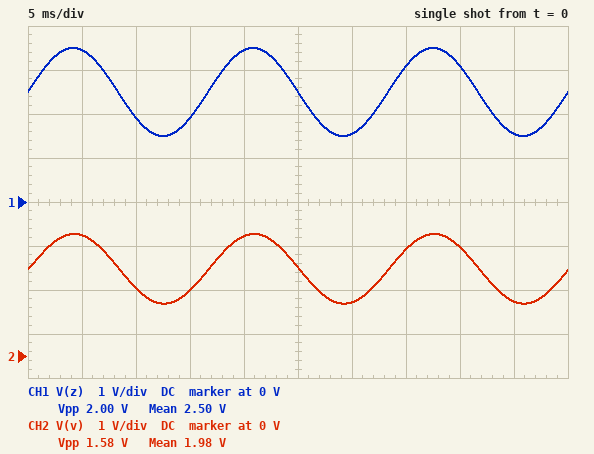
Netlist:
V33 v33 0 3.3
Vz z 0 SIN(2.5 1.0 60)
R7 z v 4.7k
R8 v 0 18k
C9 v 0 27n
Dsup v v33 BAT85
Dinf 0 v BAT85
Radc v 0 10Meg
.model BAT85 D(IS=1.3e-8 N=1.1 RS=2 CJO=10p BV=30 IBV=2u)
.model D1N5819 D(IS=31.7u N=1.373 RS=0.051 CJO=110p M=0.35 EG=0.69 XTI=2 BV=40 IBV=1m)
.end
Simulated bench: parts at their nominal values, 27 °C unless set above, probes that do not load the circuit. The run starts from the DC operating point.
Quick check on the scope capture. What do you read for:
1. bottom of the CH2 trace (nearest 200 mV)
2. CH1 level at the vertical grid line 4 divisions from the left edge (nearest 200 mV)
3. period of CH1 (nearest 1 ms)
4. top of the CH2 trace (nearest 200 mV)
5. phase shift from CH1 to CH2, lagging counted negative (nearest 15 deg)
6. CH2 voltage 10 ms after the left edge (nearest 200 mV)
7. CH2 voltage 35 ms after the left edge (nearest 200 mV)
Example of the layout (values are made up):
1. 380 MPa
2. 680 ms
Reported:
1. 1.2 V
2. 3.4 V
3. 17 ms
4. 2.8 V
5. 0 deg
6. 1.6 V
7. 2.4 V
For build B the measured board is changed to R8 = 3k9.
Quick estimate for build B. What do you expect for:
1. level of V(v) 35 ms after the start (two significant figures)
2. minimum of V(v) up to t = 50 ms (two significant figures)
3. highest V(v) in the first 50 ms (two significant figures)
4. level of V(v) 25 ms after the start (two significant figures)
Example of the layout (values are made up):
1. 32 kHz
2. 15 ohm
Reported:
1. 1.4 V
2. 680 mV
3. 1.6 V
4. 1.1 V
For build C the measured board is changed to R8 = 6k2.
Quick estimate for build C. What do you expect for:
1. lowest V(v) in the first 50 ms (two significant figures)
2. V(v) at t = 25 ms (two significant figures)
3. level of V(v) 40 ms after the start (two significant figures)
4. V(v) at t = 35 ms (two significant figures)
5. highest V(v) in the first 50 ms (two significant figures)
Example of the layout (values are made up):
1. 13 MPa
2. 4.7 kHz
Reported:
1. 850 mV
2. 1.4 V
3. 1.8 V
4. 1.7 V
5. 2.0 V
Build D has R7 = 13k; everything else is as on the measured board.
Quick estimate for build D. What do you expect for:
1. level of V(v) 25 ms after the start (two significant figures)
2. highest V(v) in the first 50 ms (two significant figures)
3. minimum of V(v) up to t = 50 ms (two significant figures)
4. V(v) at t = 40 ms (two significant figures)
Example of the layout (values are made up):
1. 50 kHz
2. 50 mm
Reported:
1. 1.5 V
2. 2.0 V
3. 870 mV
4. 1.8 V
